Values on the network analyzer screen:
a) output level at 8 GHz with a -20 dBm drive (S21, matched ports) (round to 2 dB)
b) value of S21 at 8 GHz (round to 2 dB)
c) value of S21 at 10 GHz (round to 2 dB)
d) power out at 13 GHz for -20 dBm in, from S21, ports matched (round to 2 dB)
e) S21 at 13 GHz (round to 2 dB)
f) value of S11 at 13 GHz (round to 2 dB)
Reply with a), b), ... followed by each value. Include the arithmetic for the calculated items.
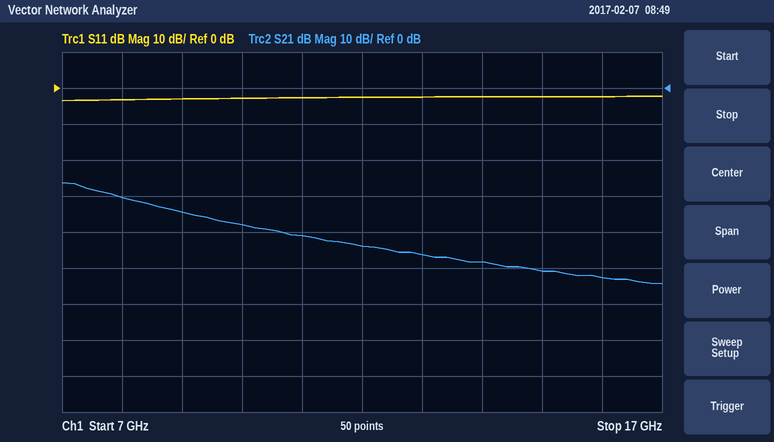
a) -20 dBm + (-30 dB) = -50 dBm
b) -30 dB
c) -38 dB
d) -20 dBm + (-46 dB) = -66 dBm
e) -46 dB
f) -2 dB
